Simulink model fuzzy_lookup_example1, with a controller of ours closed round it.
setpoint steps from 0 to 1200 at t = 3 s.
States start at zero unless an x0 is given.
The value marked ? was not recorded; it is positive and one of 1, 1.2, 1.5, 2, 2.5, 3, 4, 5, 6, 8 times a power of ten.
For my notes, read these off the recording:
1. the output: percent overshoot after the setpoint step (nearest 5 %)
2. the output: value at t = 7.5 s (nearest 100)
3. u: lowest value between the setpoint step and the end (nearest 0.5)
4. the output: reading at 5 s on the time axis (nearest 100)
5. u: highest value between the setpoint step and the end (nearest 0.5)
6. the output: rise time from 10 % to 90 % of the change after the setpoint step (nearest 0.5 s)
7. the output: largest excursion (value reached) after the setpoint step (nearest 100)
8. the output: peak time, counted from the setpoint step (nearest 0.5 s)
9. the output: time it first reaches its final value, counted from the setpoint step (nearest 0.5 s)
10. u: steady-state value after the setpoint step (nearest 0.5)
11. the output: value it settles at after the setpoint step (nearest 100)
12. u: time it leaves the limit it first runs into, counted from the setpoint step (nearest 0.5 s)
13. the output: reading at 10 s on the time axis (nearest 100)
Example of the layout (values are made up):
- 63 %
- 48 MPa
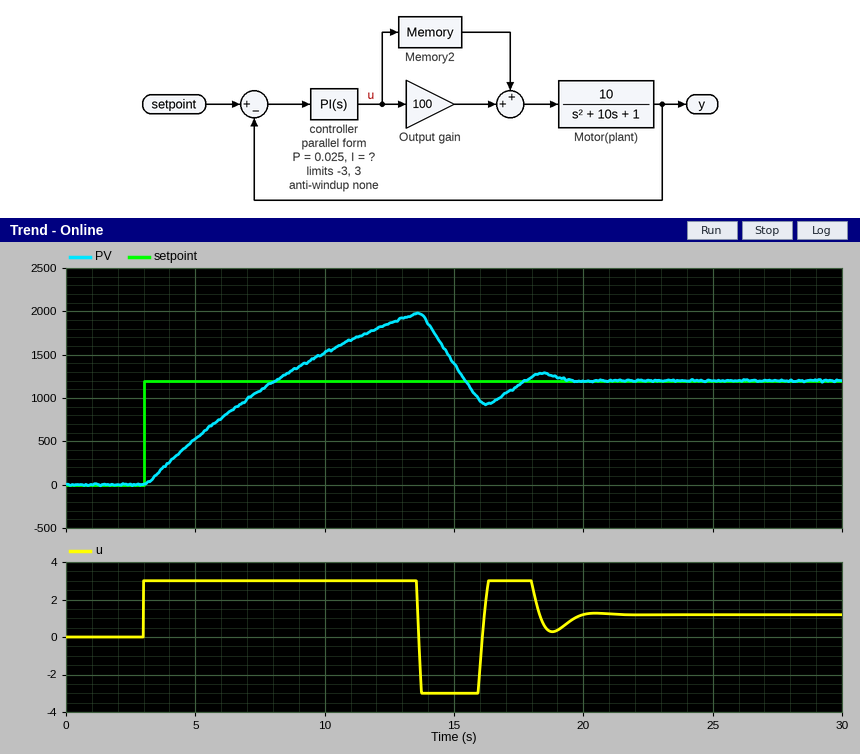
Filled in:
- 65 %
- 1100
- -3.0
- 500
- 3.0
- 4.0 s
- 2000
- 10.5 s
- 5.0 s
- 1.0
- 1200
- 10.5 s
- 1500
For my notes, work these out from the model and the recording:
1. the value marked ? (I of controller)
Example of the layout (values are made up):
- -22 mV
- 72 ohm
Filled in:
- 0.04
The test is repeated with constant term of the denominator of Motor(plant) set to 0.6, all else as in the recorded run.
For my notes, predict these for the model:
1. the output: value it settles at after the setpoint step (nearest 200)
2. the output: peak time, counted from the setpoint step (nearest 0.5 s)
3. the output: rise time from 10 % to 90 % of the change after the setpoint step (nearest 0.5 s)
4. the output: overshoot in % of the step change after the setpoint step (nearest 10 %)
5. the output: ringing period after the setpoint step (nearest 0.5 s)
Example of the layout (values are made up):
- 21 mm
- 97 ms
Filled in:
- 1200
- 9.0 s
- 3.5 s
- 80 %
- 6.5 s
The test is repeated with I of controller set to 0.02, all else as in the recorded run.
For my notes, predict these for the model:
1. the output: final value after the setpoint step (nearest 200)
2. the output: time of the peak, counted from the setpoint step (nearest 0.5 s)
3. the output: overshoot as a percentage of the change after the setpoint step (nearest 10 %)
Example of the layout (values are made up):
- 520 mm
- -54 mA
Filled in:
- 1200
- 10.0 s
- 60 %
